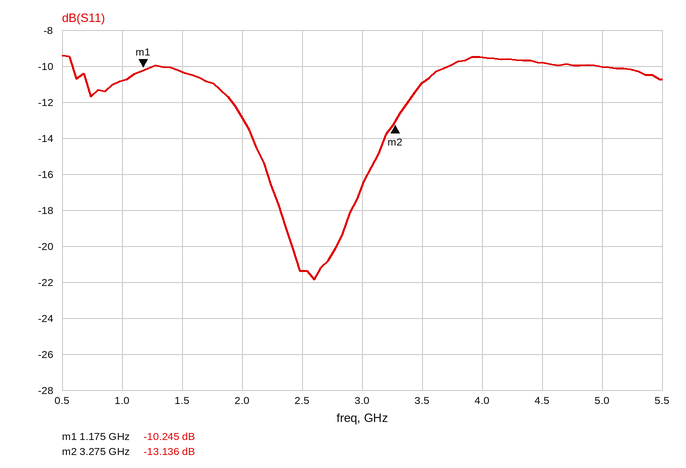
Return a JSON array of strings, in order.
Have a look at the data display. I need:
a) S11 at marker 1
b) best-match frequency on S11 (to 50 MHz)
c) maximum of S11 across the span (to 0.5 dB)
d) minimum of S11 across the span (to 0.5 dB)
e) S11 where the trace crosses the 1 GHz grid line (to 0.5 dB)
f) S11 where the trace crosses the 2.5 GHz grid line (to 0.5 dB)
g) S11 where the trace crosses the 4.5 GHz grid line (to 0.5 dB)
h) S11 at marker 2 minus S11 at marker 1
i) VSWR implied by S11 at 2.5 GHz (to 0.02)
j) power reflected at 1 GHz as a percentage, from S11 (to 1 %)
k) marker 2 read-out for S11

["-10.245 dB", "2.60 GHz", "-9.5 dB", "-22.0 dB", "-11.0 dB", "-21.5 dB", "-10.0 dB", "-2.891 dB", "1.18", "8 %", "-13.136 dB"]
